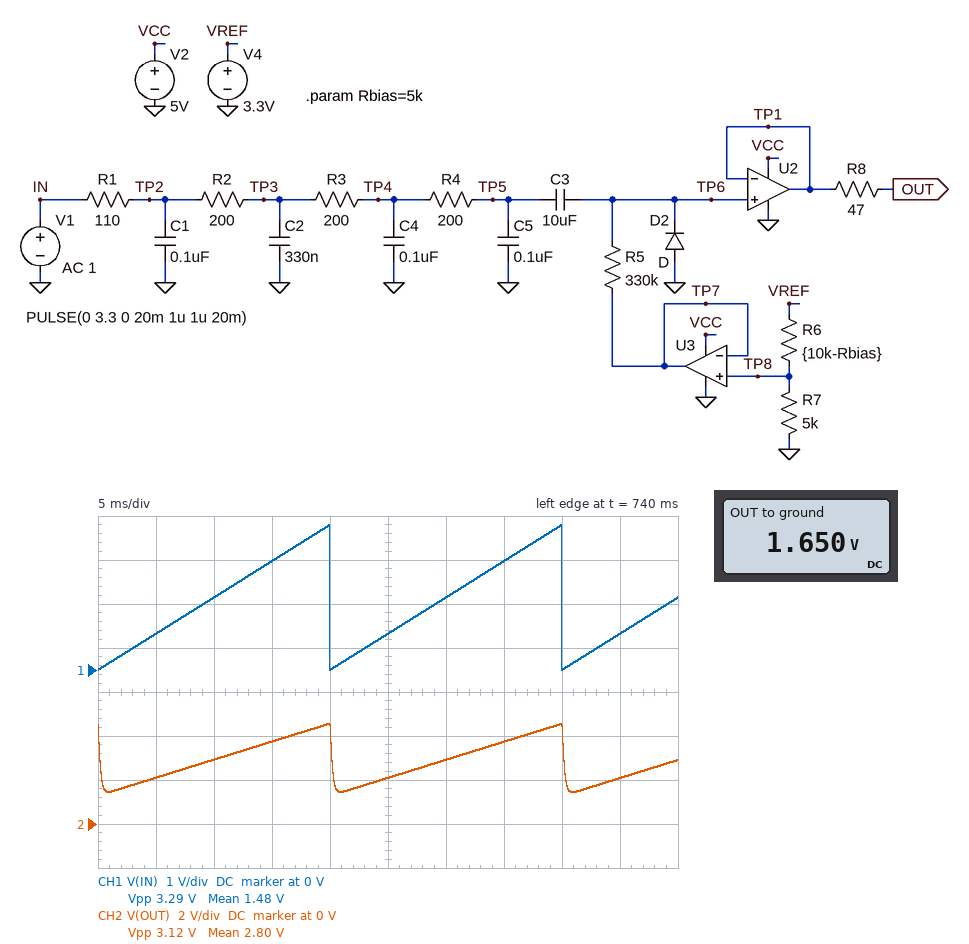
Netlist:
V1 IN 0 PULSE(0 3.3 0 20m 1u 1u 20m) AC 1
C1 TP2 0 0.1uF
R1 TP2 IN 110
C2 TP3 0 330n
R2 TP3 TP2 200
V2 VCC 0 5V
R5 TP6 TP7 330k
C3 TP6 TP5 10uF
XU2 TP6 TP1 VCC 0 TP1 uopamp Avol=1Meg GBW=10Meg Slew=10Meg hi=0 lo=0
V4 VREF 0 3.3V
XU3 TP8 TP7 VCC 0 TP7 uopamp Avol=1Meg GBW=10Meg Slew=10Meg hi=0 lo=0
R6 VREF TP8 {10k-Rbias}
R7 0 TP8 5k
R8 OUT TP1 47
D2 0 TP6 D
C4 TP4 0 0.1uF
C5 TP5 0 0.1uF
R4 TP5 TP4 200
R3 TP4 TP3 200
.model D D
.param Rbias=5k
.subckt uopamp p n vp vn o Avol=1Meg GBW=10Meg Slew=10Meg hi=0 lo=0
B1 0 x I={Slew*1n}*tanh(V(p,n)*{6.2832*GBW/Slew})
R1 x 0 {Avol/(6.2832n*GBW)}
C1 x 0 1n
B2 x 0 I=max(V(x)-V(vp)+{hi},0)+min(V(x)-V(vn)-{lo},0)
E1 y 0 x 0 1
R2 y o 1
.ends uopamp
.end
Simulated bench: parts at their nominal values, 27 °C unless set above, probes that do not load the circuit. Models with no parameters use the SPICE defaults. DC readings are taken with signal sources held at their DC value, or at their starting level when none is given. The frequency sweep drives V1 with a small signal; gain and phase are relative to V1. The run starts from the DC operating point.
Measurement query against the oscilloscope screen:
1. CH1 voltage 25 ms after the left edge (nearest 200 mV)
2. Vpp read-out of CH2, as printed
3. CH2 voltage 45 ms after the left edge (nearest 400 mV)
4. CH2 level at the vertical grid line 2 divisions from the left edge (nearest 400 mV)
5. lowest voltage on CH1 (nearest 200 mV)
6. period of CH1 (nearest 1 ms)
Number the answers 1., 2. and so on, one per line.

1. 800 mV
2. 3.12 V
3. 2.0 V
4. 2.8 V
5. 0 V
6. 20 ms
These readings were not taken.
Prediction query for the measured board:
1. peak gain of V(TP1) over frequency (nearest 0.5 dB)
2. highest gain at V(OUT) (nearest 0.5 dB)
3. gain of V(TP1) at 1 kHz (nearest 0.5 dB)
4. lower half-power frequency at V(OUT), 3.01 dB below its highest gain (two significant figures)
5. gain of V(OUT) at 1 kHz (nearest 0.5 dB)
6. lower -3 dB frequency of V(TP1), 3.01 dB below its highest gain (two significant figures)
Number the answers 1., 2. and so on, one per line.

1. 0 dB
2. 0 dB
3. -4.0 dB
4. 48 mHz
5. -4.0 dB
6. 48 mHz
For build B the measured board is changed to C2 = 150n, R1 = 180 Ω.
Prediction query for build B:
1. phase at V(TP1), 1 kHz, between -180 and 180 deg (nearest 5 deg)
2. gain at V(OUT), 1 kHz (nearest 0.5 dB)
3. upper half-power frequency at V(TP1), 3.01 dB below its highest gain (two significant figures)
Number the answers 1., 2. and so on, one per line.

1. -60 deg
2. -3.5 dB
3. 900 Hz
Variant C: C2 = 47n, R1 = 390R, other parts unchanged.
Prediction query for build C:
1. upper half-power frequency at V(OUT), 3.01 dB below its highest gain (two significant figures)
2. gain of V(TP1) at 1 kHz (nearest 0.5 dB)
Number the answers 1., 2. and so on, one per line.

1. 750 Hz
2. -4.5 dB
